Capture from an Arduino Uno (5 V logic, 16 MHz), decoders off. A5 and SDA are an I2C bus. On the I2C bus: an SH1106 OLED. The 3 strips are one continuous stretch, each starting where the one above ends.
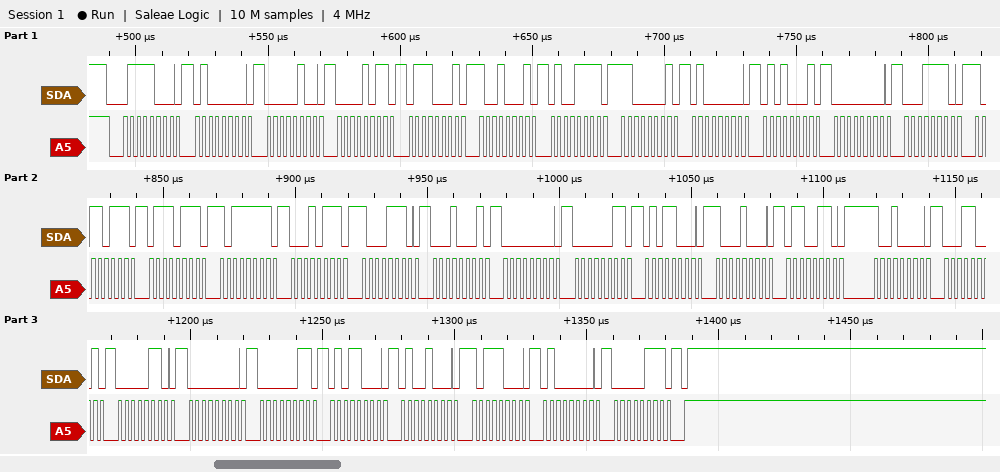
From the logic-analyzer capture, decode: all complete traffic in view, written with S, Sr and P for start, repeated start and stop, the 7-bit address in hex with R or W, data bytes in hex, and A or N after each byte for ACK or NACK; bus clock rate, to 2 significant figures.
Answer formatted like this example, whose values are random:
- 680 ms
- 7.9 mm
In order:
- S 3CW A 40 A 04 A 0B A 71 A 91 A 4F A C1 A 40 A 51 A 00 A 1E A B7 A 77 A BF A 17 A 8E A 11 A 00 A 03 A 58 A 88 A 66 A 90 A 19 A 06 A 00 A 03 A 58 A 48 A B8 A 40 A 07 A P
- 400 kHz
